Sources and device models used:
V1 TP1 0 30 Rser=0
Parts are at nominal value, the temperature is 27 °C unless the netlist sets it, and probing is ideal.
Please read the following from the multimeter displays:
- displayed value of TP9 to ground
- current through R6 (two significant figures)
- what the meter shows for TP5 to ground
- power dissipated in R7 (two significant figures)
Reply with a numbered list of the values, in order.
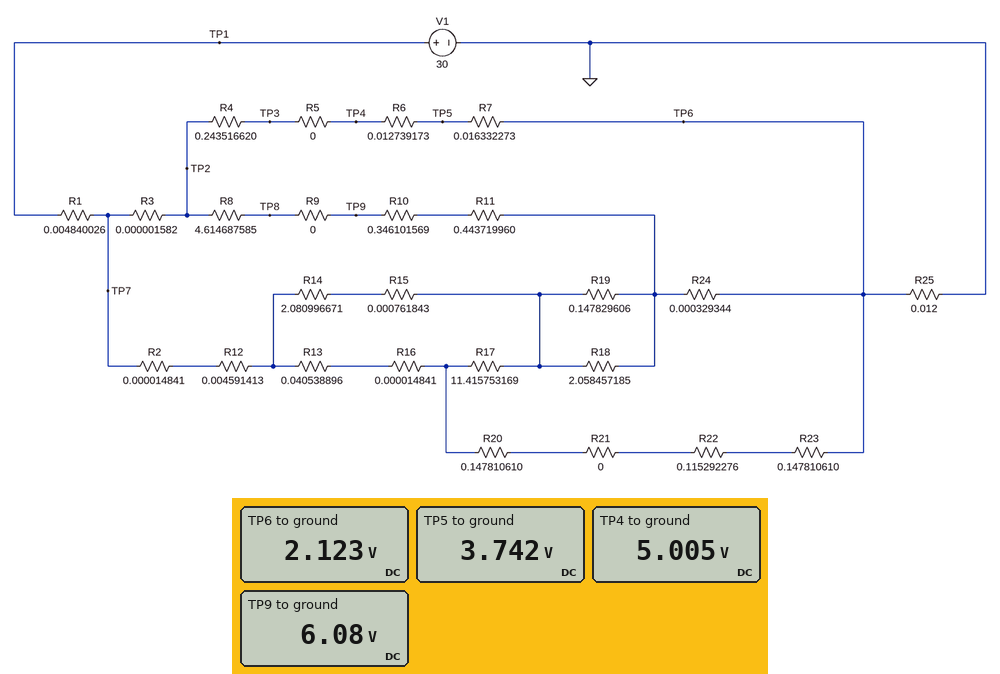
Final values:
1. 6.08 V
2. 99 A
3. 3.742 V
4. 160 W
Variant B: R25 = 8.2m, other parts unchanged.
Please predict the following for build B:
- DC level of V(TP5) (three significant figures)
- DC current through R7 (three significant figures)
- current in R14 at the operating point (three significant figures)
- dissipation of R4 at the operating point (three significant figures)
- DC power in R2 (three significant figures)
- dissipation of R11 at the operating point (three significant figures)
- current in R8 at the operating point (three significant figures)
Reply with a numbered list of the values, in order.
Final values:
1. 3.14 V
2. 101 A
3. 12.2 A
4. 2.50 kW
5. 82.3 mW
6. 11.6 W
7. 5.11 A
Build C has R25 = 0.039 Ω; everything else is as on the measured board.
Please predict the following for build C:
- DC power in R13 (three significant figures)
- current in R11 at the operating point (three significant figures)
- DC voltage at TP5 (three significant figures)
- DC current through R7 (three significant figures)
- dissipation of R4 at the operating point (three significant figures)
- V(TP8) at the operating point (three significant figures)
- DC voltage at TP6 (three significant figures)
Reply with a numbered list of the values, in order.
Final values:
1. 112 W
2. 4.31 A
3. 7.35 V
4. 85.5 A
5. 1.78 kW
6. 9.36 V
7. 5.95 V
